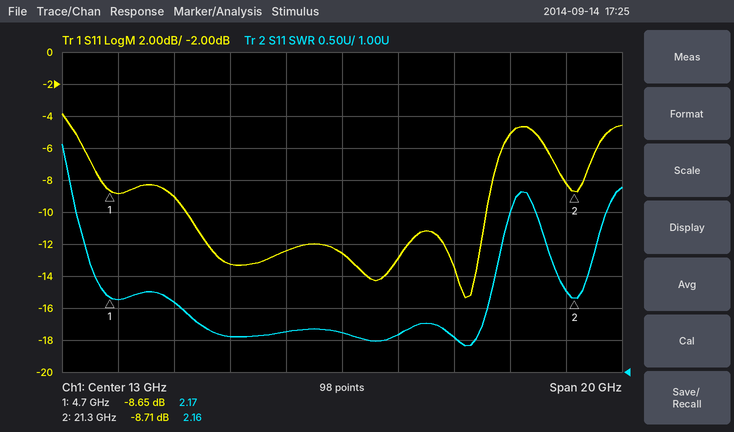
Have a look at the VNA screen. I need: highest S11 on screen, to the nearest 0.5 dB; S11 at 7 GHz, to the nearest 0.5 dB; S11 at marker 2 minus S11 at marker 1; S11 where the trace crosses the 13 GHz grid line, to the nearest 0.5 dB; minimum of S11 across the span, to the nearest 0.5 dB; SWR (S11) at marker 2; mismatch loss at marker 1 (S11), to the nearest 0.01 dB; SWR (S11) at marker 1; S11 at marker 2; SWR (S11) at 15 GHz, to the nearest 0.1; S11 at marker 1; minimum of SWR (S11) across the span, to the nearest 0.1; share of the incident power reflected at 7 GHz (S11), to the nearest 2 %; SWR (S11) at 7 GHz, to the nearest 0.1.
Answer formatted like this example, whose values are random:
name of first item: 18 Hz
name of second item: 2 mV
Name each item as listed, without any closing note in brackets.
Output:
highest S11 on screen, to the nearest 0.5 dB: -4.0 dB
S11 at 7 GHz, to the nearest 0.5 dB: -9.0 dB
S11 at marker 2 minus S11 at marker 1: -0.06 dB
S11 where the trace crosses the 13 GHz grid line, to the nearest 0.5 dB: -12.5 dB
minimum of S11 across the span, to the nearest 0.5 dB: -15.5 dB
SWR (S11) at marker 2: 2.16
mismatch loss at marker 1 (S11), to the nearest 0.01 dB: 0.64 dB
SWR (S11) at marker 1: 2.17
S11 at marker 2: -8.71 dB
SWR (S11) at 15 GHz, to the nearest 0.1: 1.6
S11 at marker 1: -8.65 dB
minimum of SWR (S11) across the span, to the nearest 0.1: 1.4
share of the incident power reflected at 7 GHz (S11), to the nearest 2 %: 12 %
SWR (S11) at 7 GHz, to the nearest 0.1: 2.1
